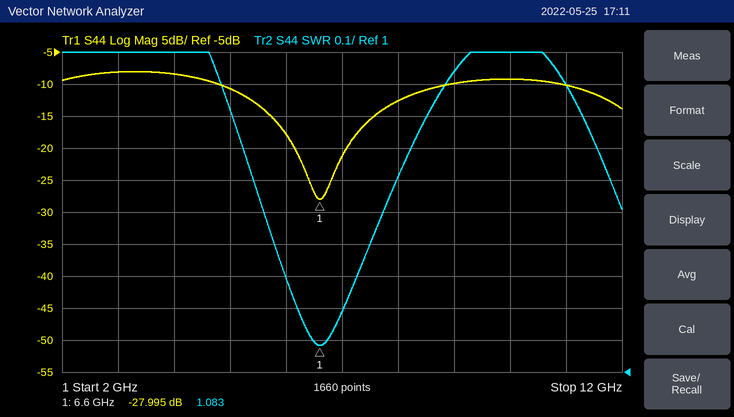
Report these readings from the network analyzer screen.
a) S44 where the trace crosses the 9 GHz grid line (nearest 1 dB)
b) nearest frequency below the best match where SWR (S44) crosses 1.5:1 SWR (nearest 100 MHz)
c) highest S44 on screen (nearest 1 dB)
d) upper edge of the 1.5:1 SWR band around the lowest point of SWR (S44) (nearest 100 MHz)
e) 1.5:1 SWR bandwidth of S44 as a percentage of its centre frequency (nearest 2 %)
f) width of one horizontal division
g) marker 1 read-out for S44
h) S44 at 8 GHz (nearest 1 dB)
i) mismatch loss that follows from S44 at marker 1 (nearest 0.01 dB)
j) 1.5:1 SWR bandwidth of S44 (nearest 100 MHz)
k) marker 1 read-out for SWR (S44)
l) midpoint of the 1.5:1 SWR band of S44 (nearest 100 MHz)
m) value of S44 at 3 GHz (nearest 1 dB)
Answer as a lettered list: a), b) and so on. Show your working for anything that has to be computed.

a) -10 dB
b) 5.6 GHz
c) -8 dB
d) 7.7 GHz
e) 2.1 GHz / 6.65 GHz ≈ 32 %
f) 1 GHz
g) -27.995 dB
h) -13 dB
i) −10 log10(1 − 10^(-27.995/10)) ≈ 0.01 dB
j) 7.7 GHz − 5.6 GHz = 2.1 GHz
k) 1.083
l) 6.7 GHz
m) -8 dB
